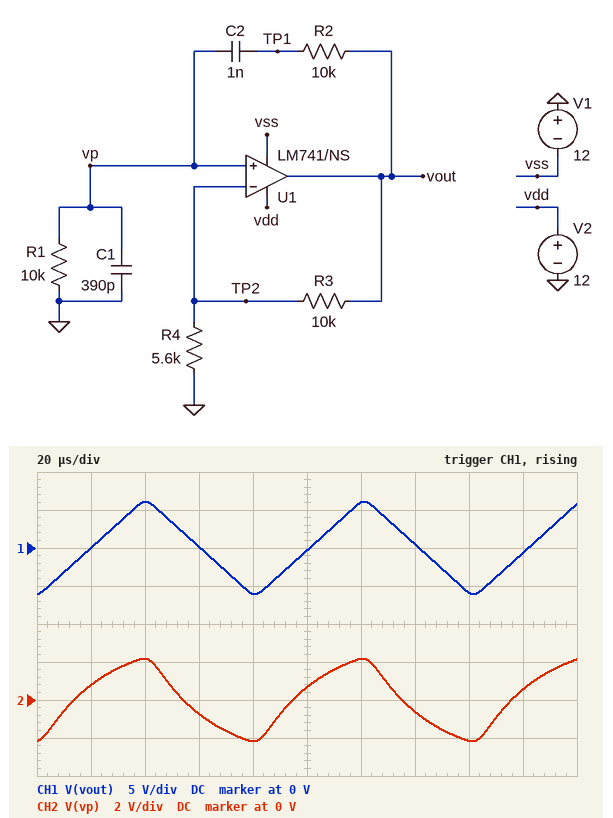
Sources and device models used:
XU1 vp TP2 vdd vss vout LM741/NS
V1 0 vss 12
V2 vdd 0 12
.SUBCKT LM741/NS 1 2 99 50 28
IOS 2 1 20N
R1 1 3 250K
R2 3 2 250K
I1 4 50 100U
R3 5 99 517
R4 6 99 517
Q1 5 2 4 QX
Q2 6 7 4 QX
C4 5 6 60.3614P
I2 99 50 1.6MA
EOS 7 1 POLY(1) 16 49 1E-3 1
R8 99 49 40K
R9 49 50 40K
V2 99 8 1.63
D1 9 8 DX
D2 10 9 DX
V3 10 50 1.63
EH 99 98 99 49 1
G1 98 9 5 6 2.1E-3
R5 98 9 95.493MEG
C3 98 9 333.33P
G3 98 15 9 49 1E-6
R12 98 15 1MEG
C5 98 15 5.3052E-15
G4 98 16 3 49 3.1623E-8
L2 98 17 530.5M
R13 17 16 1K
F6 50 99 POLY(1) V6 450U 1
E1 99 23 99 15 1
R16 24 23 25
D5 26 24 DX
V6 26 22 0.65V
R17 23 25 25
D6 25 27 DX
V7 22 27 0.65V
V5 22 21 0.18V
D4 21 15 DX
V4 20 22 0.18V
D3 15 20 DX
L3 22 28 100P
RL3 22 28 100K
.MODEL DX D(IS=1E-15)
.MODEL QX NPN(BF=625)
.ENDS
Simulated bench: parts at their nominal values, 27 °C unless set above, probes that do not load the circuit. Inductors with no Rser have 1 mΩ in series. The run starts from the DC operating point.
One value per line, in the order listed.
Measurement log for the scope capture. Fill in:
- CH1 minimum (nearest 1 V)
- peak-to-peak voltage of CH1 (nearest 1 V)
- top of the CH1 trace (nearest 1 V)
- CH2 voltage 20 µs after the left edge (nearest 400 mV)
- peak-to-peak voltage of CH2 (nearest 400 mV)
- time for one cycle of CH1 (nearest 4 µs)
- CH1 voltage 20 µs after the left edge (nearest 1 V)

-6 V
12 V
6 V
800 mV
4.4 V
80 µs
0 V
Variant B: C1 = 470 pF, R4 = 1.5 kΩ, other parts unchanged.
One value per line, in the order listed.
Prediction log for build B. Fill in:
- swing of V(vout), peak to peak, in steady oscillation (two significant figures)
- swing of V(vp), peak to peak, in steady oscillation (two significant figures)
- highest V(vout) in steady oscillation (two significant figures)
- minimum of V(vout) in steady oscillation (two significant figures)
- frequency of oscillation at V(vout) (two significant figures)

22 V
5.9 V
11 V
-11 V
5.7 kHz
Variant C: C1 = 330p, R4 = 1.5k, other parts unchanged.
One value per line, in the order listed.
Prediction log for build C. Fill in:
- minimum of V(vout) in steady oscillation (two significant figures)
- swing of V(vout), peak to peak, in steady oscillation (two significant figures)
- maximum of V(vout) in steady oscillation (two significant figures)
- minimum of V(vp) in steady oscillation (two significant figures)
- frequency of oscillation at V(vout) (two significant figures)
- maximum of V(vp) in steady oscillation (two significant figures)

-11 V
22 V
11 V
-3.0 V
5.8 kHz
3.0 V
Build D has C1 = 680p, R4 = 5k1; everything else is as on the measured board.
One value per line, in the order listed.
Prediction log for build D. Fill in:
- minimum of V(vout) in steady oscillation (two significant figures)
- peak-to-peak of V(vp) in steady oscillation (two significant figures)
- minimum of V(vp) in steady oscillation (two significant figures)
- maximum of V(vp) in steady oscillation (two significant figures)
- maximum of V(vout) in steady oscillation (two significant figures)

-6.0 V
4.0 V
-2.0 V
2.0 V
6.0 V
